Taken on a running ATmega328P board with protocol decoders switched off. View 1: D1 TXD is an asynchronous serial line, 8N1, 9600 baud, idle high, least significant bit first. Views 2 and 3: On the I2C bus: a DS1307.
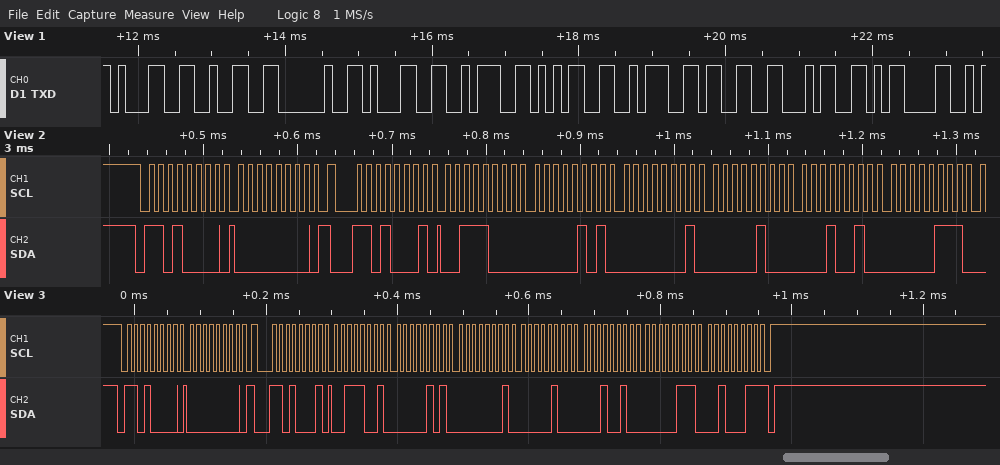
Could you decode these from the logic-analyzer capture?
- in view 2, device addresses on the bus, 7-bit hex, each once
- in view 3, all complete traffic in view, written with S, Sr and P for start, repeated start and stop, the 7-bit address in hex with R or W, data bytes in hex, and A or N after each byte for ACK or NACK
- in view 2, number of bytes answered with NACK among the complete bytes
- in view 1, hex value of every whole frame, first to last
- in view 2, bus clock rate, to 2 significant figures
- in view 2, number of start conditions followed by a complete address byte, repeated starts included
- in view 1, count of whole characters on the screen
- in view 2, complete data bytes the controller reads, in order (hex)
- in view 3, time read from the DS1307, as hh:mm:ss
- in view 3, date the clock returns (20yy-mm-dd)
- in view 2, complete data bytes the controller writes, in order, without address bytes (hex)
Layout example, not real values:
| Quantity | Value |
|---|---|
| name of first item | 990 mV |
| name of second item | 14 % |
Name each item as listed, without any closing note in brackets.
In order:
| Quantity | Value |
|---|---|
| in view 2, device addresses on the bus, 7-bit hex, each once | 0x68 |
| in view 3, all complete traffic in view, written with S, Sr and P for start, repeated start and stop, the 7-bit address in hex with R or W, data bytes in hex, and A or N after each byte for ACK or NACK | S 68W A 00 A Sr 68R A 39 A 05 A 01 A 04 A 12 A 07 A 23 N P |
| in view 2, number of bytes answered with NACK among the complete bytes | 0 |
| in view 1, hex value of every whole frame, first to last | 31 32 20 31 3A 35 3A 33 34 0D |
| in view 2, bus clock rate, to 2 significant figures | 100 kHz |
| in view 2, number of start conditions followed by a complete address byte, repeated starts included | 2 |
| in view 1, count of whole characters on the screen | 10 |
| in view 2, complete data bytes the controller reads, in order | 38 05 01 04 12 07 |
| in view 3, time read from the DS1307, as hh:mm:ss | 01:05:39 |
| in view 3, date the clock returns | 2023-07-12 |
| in view 2, complete data bytes the controller writes, in order, without address bytes | 00 |
